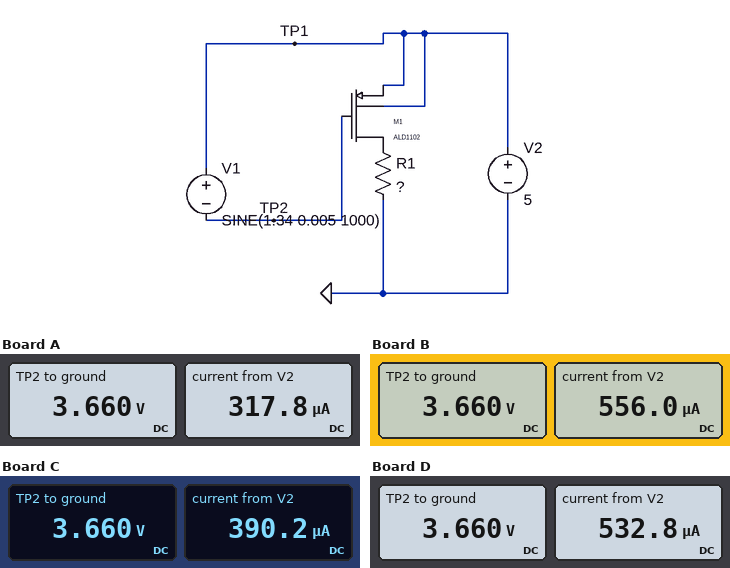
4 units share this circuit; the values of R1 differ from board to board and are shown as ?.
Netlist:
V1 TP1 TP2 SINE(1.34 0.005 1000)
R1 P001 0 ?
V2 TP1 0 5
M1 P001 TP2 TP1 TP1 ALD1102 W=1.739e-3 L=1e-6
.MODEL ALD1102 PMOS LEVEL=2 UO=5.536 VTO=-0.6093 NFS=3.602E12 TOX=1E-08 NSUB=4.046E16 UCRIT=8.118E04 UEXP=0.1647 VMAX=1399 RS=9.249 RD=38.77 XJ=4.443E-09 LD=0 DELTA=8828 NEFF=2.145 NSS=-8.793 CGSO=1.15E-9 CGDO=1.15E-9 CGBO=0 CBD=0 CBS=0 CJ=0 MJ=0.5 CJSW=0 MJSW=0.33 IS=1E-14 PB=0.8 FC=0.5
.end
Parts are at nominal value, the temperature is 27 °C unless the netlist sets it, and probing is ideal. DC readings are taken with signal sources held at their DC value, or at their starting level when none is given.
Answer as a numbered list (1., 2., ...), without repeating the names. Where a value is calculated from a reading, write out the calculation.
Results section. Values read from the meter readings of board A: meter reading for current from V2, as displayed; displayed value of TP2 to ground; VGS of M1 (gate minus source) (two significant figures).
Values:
1. 317.8 µA
2. 3.660 V
3. 3.66 V - 5 V = -1.3 V
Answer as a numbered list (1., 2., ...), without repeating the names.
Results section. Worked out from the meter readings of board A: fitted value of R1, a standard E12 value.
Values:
1. 15 kΩ
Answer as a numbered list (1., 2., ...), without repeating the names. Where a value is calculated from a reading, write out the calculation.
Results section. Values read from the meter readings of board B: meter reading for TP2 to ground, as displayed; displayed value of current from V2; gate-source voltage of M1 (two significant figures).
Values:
1. 3.660 V
2. 556.0 µA
3. 3.66 V - 5 V = -1.3 V
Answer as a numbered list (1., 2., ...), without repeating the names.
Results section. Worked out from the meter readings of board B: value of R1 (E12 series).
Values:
1. 3.9 kΩ
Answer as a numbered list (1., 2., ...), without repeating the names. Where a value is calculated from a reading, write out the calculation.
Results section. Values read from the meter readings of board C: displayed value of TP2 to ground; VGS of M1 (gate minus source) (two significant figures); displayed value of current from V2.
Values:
1. 3.660 V
2. 3.66 V - 5 V = -1.3 V
3. 390.2 µA
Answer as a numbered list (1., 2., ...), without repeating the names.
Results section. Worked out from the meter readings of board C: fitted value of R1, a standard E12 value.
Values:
1. 12 kΩ
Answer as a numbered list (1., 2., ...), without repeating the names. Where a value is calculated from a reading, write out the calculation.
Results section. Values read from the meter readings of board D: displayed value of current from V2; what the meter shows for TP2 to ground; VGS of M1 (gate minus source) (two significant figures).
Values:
1. 532.8 µA
2. 3.660 V
3. 3.66 V - 5 V = -1.3 V
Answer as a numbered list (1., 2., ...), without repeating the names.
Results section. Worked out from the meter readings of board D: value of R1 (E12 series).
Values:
1. 5.6 kΩ
